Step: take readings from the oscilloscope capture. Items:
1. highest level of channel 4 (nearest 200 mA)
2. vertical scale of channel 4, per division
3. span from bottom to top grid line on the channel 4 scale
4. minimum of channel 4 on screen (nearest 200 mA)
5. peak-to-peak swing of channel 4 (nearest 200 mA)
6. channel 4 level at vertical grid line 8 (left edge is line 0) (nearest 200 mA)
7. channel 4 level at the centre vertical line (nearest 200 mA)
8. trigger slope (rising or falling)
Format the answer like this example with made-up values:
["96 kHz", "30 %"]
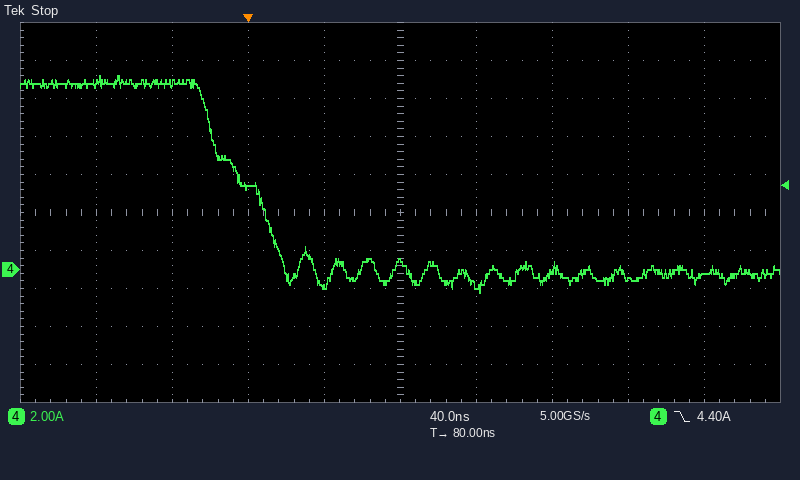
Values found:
["10.2 A", "2 A", "20 A", "-1.2 A", "11.4 A", "-400 mA", "400 mA", "falling"]
